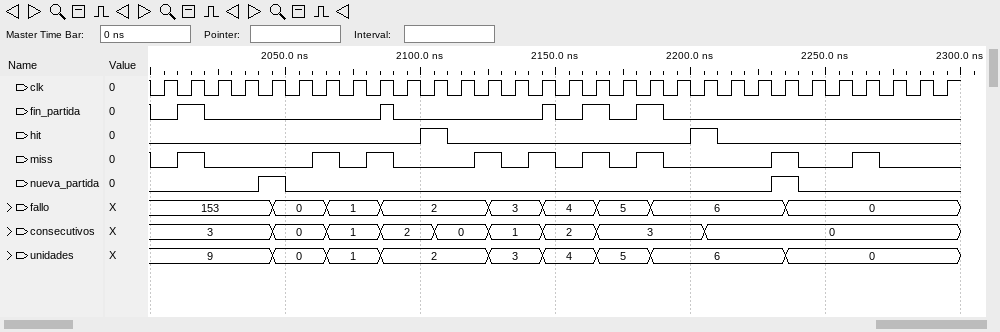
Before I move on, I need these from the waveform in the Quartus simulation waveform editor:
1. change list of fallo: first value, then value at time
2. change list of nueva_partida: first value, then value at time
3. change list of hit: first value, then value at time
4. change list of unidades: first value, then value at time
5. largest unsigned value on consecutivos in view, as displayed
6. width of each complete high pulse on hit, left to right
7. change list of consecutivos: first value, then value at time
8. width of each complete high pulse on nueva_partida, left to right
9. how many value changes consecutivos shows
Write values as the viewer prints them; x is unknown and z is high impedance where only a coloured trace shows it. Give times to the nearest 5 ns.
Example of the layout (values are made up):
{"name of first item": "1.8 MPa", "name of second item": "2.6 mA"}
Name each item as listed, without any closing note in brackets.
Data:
{"change list of fallo: first value, then value at time": "153, 0 at 2045 ns, 1 at 2065 ns, 2 at 2085 ns, 3 at 2125 ns, 4 at 2145 ns, 5 at 2165 ns, 6 at 2185 ns, 0 at 2235 ns", "change list of nueva_partida: first value, then value at time": "0, 1 at 2040 ns, 0 at 2050 ns, 1 at 2230 ns, 0 at 2240 ns", "change list of hit: first value, then value at time": "0, 1 at 2100 ns, 0 at 2110 ns, 1 at 2200 ns, 0 at 2210 ns", "change list of unidades: first value, then value at time": "9, 0 at 2045 ns, 1 at 2065 ns, 2 at 2085 ns, 3 at 2125 ns, 4 at 2145 ns, 5 at 2165 ns, 6 at 2185 ns, 0 at 2235 ns", "largest unsigned value on consecutivos in view, as displayed": "3", "width of each complete high pulse on hit, left to right": "10 ns, 10 ns", "change list of consecutivos: first value, then value at time": "3, 0 at 2045 ns, 1 at 2065 ns, 2 at 2085 ns, 0 at 2105 ns, 1 at 2125 ns, 2 at 2145 ns, 3 at 2165 ns, 0 at 2205 ns", "width of each complete high pulse on nueva_partida, left to right": "10 ns, 10 ns", "how many value changes consecutivos shows": "8"}
